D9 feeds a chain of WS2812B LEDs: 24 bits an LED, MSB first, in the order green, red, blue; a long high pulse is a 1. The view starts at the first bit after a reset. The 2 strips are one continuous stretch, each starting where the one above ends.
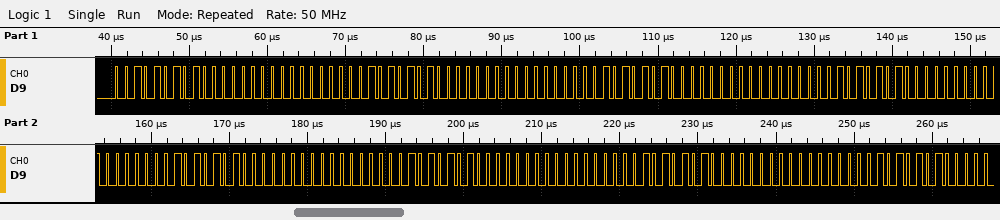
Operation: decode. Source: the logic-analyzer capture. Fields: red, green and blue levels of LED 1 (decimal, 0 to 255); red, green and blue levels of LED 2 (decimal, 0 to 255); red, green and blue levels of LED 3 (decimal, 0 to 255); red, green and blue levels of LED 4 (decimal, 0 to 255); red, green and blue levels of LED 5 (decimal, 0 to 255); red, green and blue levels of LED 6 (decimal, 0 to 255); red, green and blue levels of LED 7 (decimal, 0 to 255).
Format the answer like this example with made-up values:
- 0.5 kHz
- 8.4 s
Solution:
- 128, 42, 0
- 128, 42, 0
- 128, 42, 0
- 128, 42, 0
- 128, 42, 0
- 128, 42, 0
- 128, 42, 0
